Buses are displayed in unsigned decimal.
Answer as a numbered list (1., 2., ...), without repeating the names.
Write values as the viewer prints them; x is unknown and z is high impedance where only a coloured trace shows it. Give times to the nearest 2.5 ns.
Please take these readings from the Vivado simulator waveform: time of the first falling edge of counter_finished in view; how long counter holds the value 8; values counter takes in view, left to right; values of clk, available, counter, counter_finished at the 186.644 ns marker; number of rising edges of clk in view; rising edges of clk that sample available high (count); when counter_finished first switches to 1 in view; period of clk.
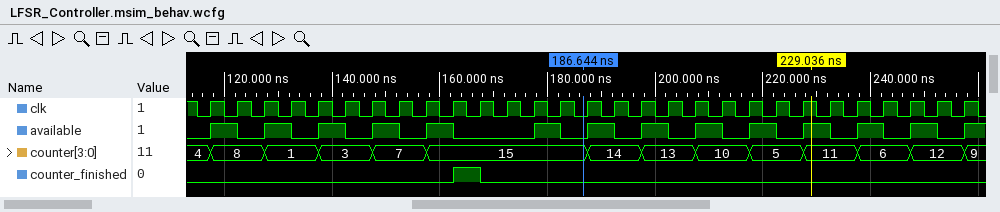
1. 167.5 ns
2. 10 ns
3. 4, 8, 1, 3, 7, 15, 14, 13, 10, 5, 11, 6, 12, 9
4. clk=0, available=0, counter=15, counter_finished=0
5. 29
6. 13
7. 162.5 ns
8. 5 ns
